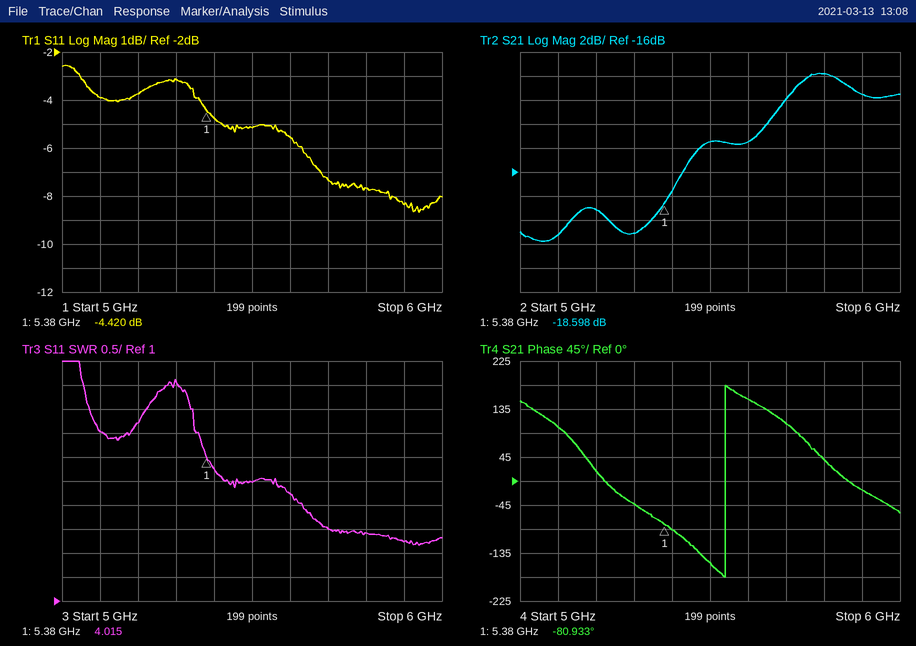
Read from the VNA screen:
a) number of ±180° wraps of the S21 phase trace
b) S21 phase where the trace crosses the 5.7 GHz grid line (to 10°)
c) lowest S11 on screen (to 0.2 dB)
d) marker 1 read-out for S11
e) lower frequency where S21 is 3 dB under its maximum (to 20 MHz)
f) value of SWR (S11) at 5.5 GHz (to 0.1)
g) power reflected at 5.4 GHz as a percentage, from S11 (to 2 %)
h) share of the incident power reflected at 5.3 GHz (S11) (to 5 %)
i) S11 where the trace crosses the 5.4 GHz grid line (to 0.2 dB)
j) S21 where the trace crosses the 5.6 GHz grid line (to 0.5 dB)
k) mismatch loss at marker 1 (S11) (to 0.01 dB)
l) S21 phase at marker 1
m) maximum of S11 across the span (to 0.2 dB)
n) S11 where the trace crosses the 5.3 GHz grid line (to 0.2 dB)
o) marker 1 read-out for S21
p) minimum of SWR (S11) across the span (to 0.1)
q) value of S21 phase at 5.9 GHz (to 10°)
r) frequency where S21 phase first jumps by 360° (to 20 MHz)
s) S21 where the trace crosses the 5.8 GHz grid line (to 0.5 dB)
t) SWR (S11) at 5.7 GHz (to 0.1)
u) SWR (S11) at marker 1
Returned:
1
110°
-8.6 dB
-4.420 dB
5.68 GHz
3.5
34 %
50 %
-4.8 dB
-13.5 dB
1.95 dB
-80.933°
-2.6 dB
-3.2 dB
-18.598 dB
2.2
-20°
5.54 GHz
-8.0 dB
2.5
4.015
